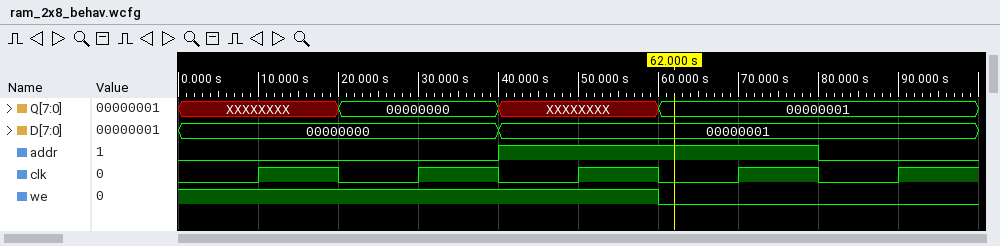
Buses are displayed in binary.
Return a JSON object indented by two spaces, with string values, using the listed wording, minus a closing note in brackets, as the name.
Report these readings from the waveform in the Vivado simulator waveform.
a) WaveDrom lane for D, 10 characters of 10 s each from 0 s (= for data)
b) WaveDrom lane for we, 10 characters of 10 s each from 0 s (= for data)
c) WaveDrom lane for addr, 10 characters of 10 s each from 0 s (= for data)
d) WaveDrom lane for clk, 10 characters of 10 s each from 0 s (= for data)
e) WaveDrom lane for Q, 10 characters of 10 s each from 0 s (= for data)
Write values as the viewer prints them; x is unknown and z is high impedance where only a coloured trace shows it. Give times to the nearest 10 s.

{
  "WaveDrom lane for D, 10 characters of 10 s each from 0 s": "{name: 'D', wave: '=...=.....', data: '00000000 00000001'}",
  "WaveDrom lane for we, 10 characters of 10 s each from 0 s": "{name: 'we', wave: '1.....0...'}",
  "WaveDrom lane for addr, 10 characters of 10 s each from 0 s": "{name: 'addr', wave: '0...1...0.'}",
  "WaveDrom lane for clk, 10 characters of 10 s each from 0 s": "{name: 'clk', wave: '0101010101'}",
  "WaveDrom lane for Q, 10 characters of 10 s each from 0 s": "{name: 'Q', wave: 'x.=.x.=...', data: '00000000 00000001'}"
}
